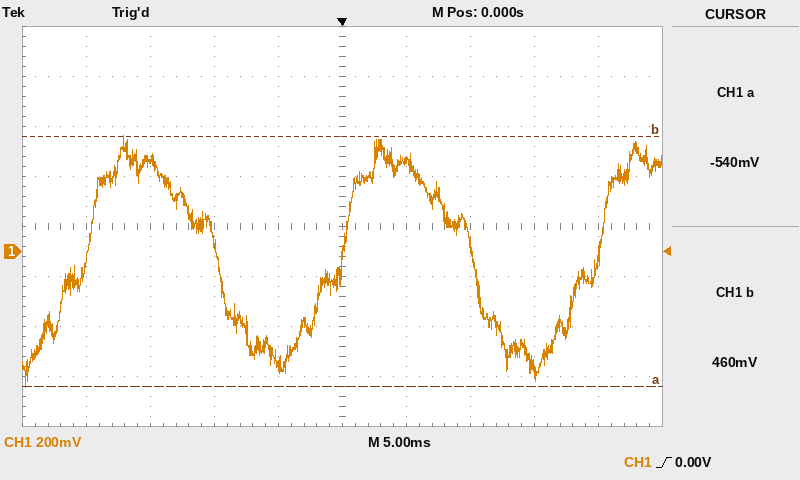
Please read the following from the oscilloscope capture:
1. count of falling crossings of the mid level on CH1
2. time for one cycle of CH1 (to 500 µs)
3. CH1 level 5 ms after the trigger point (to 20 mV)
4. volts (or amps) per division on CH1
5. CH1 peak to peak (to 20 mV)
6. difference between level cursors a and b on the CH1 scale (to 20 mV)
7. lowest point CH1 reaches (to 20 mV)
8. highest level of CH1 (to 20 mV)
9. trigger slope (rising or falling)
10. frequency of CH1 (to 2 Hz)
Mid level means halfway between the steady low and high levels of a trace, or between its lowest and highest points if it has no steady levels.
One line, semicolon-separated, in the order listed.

2; 20.0 ms; 360 mV; 200 mV; 1.00 V; 1.00 V; -540 mV; 460 mV; rising; 50 Hz
